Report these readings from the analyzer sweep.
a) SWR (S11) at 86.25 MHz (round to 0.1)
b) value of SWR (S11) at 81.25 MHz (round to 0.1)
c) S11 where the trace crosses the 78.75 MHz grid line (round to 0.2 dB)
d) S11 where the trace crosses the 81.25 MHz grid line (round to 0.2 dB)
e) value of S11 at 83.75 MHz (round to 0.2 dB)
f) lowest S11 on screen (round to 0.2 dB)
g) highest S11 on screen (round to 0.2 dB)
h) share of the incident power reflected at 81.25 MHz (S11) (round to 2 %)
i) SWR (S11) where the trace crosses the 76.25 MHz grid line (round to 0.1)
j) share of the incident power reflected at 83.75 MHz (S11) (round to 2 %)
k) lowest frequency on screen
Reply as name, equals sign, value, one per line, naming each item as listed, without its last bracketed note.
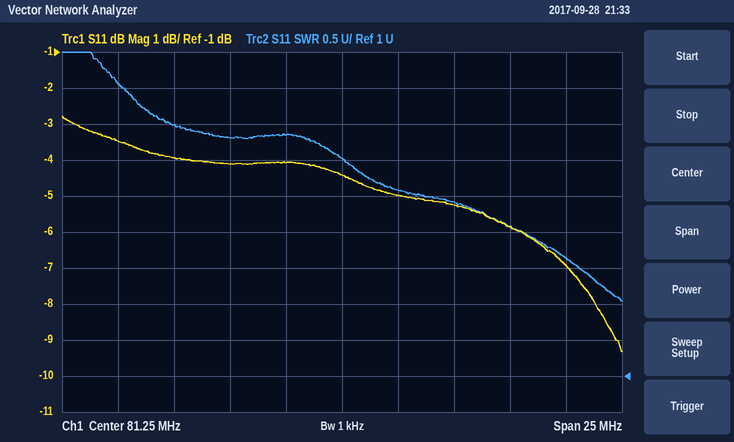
SWR (S11) at 86.25 MHz = 3.4
value of SWR (S11) at 81.25 MHz = 4.0
S11 where the trace crosses the 78.75 MHz grid line = -4.0 dB
S11 where the trace crosses the 81.25 MHz grid line = -4.4 dB
value of S11 at 83.75 MHz = -5.0 dB
lowest S11 on screen = -9.4 dB
highest S11 on screen = -2.8 dB
share of the incident power reflected at 81.25 MHz (S11) = 36 %
SWR (S11) where the trace crosses the 76.25 MHz grid line = 4.3
share of the incident power reflected at 83.75 MHz (S11) = 32 %
lowest frequency on screen = 68.75 MHz
